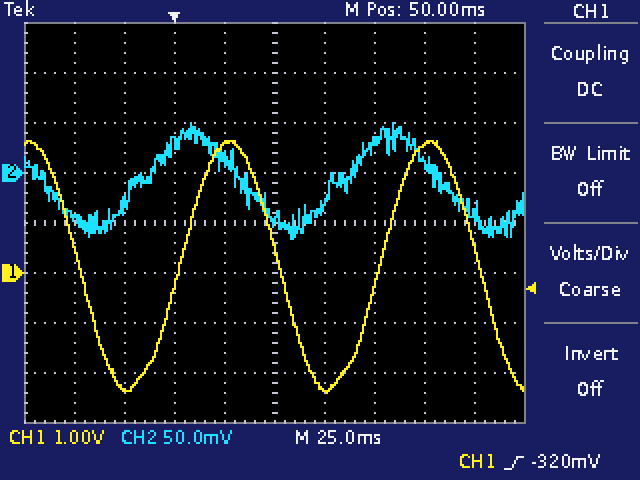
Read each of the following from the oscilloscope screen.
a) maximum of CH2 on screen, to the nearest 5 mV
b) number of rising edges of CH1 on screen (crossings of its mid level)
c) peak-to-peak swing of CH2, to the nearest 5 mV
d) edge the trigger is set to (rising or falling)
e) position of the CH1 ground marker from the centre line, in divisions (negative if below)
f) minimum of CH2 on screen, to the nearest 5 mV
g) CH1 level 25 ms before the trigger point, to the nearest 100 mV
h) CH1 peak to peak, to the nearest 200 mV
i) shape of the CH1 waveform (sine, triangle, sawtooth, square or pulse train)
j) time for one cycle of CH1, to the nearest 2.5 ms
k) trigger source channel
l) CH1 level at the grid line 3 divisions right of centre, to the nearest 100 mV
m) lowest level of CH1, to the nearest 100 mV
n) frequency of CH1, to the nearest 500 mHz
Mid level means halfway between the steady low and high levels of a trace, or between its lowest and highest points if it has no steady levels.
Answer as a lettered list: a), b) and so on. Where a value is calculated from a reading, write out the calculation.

a) 50 mV
b) 2
c) 50 mV − (-65 mV) = 115 mV
d) rising
e) -1.0 div
f) -65 mV
g) -2.3 V
h) 5.0 V
i) sine
j) 100.0 ms
k) CH1
l) 2.6 V
m) -2.4 V
n) 1 / 100.0 ms ≈ 10.0 Hz
